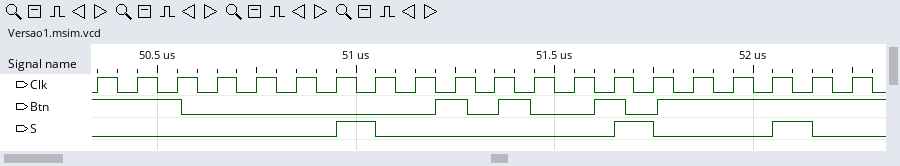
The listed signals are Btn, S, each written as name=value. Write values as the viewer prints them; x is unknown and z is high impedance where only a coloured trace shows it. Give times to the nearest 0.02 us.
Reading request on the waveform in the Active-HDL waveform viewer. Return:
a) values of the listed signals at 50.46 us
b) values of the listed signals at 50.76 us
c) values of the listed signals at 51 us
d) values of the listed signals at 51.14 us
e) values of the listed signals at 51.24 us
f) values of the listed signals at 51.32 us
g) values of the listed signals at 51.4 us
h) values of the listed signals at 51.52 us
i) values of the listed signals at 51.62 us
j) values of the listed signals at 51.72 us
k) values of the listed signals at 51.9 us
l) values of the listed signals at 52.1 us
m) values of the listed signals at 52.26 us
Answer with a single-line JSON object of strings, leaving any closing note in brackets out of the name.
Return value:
{"values of the listed signals at 50.46 us": "Btn=1, S=0", "values of the listed signals at 50.76 us": "Btn=0, S=0", "values of the listed signals at 51 us": "Btn=0, S=1", "values of the listed signals at 51.14 us": "Btn=0, S=0", "values of the listed signals at 51.24 us": "Btn=1, S=0", "values of the listed signals at 51.32 us": "Btn=0, S=0", "values of the listed signals at 51.4 us": "Btn=1, S=0", "values of the listed signals at 51.52 us": "Btn=0, S=0", "values of the listed signals at 51.62 us": "Btn=1, S=0", "values of the listed signals at 51.72 us": "Btn=0, S=1", "values of the listed signals at 51.9 us": "Btn=1, S=0", "values of the listed signals at 52.1 us": "Btn=1, S=1", "values of the listed signals at 52.26 us": "Btn=1, S=0"}
